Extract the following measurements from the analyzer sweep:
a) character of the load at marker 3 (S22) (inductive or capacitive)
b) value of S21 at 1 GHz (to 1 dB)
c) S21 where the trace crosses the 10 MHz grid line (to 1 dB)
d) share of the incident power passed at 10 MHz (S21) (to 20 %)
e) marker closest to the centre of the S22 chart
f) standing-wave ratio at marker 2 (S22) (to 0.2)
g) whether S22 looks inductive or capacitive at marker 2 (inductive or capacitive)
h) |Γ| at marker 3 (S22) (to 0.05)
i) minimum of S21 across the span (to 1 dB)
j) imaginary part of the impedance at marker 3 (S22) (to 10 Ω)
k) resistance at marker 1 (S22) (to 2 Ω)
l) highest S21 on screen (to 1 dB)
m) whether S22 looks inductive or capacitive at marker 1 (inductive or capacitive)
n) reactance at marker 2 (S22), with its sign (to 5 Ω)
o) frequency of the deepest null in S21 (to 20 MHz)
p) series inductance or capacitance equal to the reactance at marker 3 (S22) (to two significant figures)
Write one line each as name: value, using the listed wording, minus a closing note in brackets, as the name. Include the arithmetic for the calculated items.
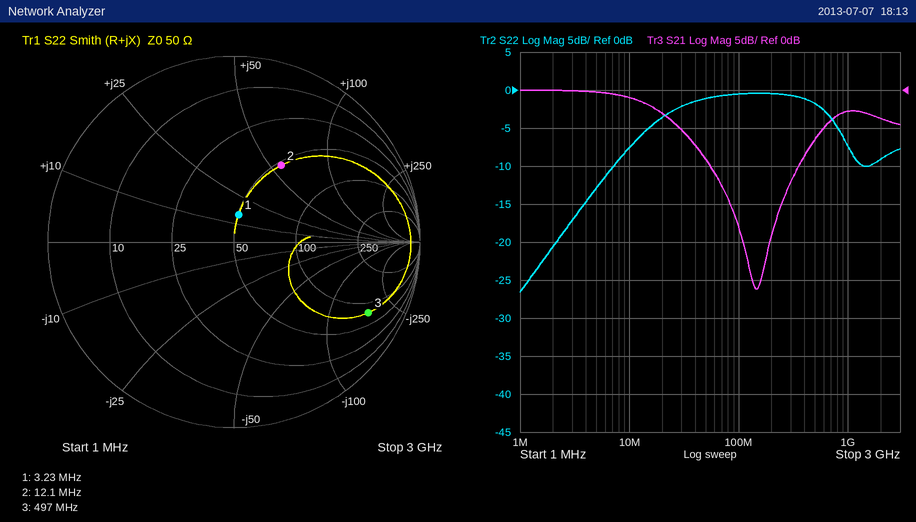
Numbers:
character of the load at marker 3 (S22): capacitive
value of S21 at 1 GHz: -3 dB
S21 where the trace crosses the 10 MHz grid line: -1 dB
share of the incident power passed at 10 MHz (S21): 10^(-1/10) ≈ 79.4 %, so 80 % to the nearest 20 %
marker closest to the centre of the S22 chart: marker 1
standing-wave ratio at marker 2 (S22): 2.8
whether S22 looks inductive or capacitive at marker 2: inductive
|Γ| at marker 3 (S22): 0.80
minimum of S21 across the span: -26 dB
imaginary part of the impedance at marker 3 (S22): -170 Ω
resistance at marker 1 (S22): 50 Ω
highest S21 on screen: 0 dB
whether S22 looks inductive or capacitive at marker 1: inductive
reactance at marker 2 (S22), with its sign: +55 Ω
frequency of the deepest null in S21: 140 MHz
series inductance or capacitance equal to the reactance at marker 3 (S22): C = 1/(2π × 497 MHz × 170 Ω) ≈ 1.9 pF
